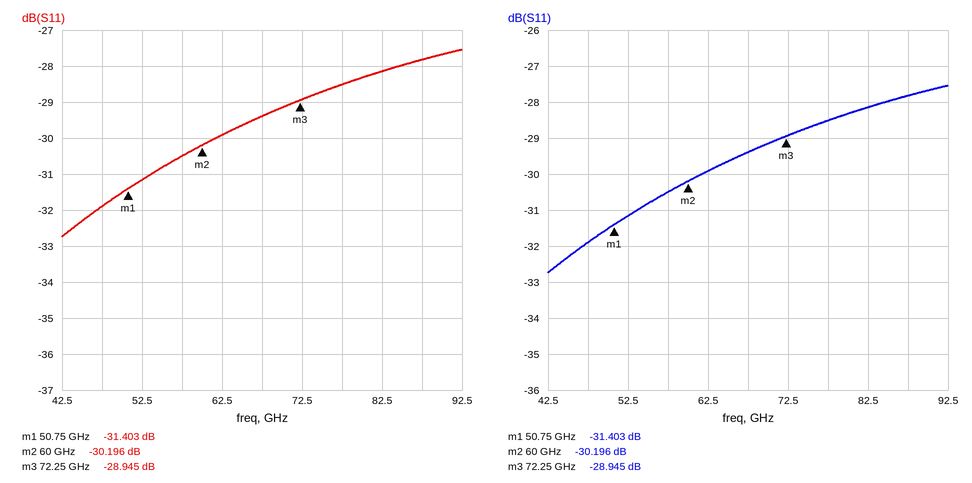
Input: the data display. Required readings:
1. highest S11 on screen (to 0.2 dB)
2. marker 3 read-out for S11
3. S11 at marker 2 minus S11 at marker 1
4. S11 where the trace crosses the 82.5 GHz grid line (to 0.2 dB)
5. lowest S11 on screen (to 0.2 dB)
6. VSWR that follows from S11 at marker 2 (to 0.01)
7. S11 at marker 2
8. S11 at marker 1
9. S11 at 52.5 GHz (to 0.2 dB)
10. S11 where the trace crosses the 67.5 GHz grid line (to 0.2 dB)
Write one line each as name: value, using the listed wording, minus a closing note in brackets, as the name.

highest S11 on screen: -27.6 dB
marker 3 read-out for S11: -28.945 dB
S11 at marker 2 minus S11 at marker 1: 1.207 dB
S11 where the trace crosses the 82.5 GHz grid line: -28.2 dB
lowest S11 on screen: -32.8 dB
VSWR that follows from S11 at marker 2: 1.06
S11 at marker 2: -30.196 dB
S11 at marker 1: -31.403 dB
S11 at 52.5 GHz: -31.2 dB
S11 where the trace crosses the 67.5 GHz grid line: -29.4 dB
